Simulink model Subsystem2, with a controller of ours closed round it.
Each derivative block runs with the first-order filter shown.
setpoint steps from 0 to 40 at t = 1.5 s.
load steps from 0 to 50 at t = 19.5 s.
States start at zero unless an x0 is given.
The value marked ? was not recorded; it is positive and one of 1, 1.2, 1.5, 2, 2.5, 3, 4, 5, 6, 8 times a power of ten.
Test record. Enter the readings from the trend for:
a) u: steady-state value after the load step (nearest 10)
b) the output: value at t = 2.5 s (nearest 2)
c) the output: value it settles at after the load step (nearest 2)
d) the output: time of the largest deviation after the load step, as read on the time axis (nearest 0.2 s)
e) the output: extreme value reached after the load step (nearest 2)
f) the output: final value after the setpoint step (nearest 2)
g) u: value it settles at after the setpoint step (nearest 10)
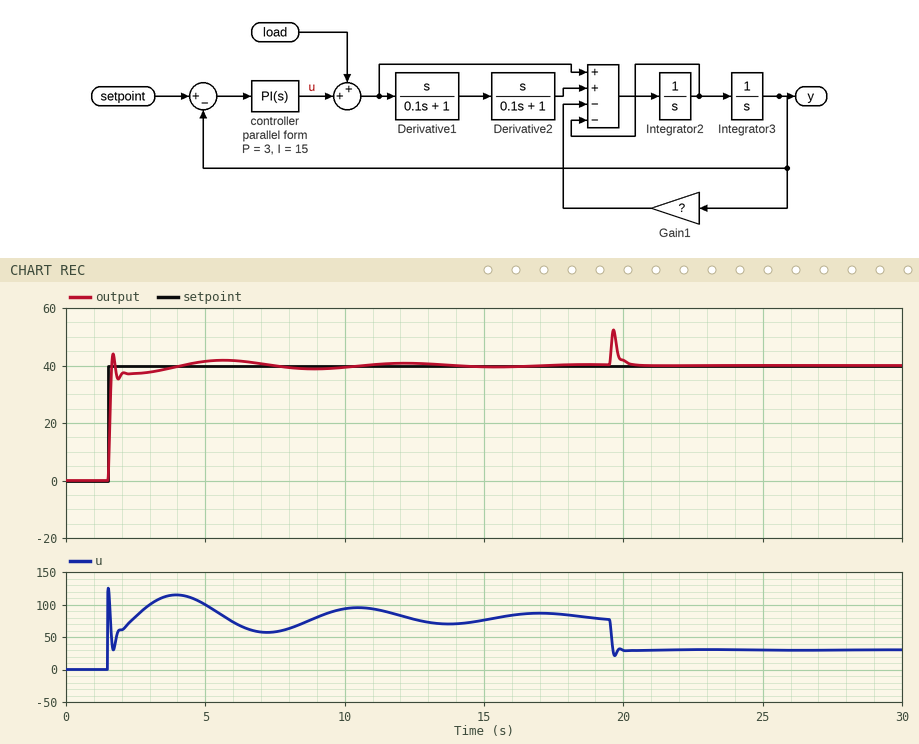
30
38
40
19.6 s
52
40
80
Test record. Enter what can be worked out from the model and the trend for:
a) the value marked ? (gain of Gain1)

2
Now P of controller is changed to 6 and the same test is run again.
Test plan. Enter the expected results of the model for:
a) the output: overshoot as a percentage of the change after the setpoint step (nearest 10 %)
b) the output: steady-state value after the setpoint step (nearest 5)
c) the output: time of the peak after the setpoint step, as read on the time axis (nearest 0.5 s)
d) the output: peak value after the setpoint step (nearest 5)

20 %
40
1.5 s
45
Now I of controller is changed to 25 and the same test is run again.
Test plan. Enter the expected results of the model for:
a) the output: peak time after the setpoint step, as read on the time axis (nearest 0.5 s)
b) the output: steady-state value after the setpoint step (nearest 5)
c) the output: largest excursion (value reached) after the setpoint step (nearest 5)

1.5 s
40
50
